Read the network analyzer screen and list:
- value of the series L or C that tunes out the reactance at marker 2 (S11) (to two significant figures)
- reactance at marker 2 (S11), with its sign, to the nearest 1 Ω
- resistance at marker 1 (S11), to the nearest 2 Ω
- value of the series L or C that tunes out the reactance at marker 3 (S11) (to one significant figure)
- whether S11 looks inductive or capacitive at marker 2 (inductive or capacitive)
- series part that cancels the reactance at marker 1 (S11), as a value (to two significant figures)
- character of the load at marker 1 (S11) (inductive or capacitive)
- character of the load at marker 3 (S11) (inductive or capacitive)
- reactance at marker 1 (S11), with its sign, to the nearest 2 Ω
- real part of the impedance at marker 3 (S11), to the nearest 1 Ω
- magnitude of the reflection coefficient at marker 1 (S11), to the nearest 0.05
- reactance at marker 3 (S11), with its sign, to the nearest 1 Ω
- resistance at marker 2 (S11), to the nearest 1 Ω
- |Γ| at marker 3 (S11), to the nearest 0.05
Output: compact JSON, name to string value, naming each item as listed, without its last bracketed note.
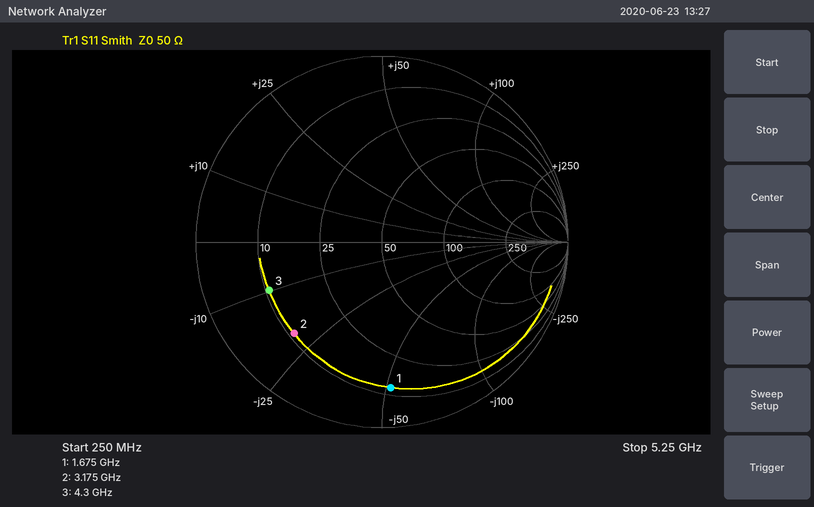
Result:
{"value of the series L or C that tunes out the reactance at marker 2 (S11)": "1.0 nH", "reactance at marker 2 (S11), with its sign, to the nearest 1 Ω": "-20 Ω", "resistance at marker 1 (S11), to the nearest 2 Ω": "12 Ω", "value of the series L or C that tunes out the reactance at marker 3 (S11)": "400 pH", "whether S11 looks inductive or capacitive at marker 2": "capacitive", "series part that cancels the reactance at marker 1 (S11), as a value": "4.9 nH", "character of the load at marker 1 (S11)": "capacitive", "character of the load at marker 3 (S11)": "capacitive", "reactance at marker 1 (S11), with its sign, to the nearest 2 Ω": "-52 Ω", "real part of the impedance at marker 3 (S11), to the nearest 1 Ω": "11 Ω", "magnitude of the reflection coefficient at marker 1 (S11), to the nearest 0.05": "0.80", "reactance at marker 3 (S11), with its sign, to the nearest 1 Ω": "-10 Ω", "resistance at marker 2 (S11), to the nearest 1 Ω": "11 Ω", "|Γ| at marker 3 (S11), to the nearest 0.05": "0.65"}
